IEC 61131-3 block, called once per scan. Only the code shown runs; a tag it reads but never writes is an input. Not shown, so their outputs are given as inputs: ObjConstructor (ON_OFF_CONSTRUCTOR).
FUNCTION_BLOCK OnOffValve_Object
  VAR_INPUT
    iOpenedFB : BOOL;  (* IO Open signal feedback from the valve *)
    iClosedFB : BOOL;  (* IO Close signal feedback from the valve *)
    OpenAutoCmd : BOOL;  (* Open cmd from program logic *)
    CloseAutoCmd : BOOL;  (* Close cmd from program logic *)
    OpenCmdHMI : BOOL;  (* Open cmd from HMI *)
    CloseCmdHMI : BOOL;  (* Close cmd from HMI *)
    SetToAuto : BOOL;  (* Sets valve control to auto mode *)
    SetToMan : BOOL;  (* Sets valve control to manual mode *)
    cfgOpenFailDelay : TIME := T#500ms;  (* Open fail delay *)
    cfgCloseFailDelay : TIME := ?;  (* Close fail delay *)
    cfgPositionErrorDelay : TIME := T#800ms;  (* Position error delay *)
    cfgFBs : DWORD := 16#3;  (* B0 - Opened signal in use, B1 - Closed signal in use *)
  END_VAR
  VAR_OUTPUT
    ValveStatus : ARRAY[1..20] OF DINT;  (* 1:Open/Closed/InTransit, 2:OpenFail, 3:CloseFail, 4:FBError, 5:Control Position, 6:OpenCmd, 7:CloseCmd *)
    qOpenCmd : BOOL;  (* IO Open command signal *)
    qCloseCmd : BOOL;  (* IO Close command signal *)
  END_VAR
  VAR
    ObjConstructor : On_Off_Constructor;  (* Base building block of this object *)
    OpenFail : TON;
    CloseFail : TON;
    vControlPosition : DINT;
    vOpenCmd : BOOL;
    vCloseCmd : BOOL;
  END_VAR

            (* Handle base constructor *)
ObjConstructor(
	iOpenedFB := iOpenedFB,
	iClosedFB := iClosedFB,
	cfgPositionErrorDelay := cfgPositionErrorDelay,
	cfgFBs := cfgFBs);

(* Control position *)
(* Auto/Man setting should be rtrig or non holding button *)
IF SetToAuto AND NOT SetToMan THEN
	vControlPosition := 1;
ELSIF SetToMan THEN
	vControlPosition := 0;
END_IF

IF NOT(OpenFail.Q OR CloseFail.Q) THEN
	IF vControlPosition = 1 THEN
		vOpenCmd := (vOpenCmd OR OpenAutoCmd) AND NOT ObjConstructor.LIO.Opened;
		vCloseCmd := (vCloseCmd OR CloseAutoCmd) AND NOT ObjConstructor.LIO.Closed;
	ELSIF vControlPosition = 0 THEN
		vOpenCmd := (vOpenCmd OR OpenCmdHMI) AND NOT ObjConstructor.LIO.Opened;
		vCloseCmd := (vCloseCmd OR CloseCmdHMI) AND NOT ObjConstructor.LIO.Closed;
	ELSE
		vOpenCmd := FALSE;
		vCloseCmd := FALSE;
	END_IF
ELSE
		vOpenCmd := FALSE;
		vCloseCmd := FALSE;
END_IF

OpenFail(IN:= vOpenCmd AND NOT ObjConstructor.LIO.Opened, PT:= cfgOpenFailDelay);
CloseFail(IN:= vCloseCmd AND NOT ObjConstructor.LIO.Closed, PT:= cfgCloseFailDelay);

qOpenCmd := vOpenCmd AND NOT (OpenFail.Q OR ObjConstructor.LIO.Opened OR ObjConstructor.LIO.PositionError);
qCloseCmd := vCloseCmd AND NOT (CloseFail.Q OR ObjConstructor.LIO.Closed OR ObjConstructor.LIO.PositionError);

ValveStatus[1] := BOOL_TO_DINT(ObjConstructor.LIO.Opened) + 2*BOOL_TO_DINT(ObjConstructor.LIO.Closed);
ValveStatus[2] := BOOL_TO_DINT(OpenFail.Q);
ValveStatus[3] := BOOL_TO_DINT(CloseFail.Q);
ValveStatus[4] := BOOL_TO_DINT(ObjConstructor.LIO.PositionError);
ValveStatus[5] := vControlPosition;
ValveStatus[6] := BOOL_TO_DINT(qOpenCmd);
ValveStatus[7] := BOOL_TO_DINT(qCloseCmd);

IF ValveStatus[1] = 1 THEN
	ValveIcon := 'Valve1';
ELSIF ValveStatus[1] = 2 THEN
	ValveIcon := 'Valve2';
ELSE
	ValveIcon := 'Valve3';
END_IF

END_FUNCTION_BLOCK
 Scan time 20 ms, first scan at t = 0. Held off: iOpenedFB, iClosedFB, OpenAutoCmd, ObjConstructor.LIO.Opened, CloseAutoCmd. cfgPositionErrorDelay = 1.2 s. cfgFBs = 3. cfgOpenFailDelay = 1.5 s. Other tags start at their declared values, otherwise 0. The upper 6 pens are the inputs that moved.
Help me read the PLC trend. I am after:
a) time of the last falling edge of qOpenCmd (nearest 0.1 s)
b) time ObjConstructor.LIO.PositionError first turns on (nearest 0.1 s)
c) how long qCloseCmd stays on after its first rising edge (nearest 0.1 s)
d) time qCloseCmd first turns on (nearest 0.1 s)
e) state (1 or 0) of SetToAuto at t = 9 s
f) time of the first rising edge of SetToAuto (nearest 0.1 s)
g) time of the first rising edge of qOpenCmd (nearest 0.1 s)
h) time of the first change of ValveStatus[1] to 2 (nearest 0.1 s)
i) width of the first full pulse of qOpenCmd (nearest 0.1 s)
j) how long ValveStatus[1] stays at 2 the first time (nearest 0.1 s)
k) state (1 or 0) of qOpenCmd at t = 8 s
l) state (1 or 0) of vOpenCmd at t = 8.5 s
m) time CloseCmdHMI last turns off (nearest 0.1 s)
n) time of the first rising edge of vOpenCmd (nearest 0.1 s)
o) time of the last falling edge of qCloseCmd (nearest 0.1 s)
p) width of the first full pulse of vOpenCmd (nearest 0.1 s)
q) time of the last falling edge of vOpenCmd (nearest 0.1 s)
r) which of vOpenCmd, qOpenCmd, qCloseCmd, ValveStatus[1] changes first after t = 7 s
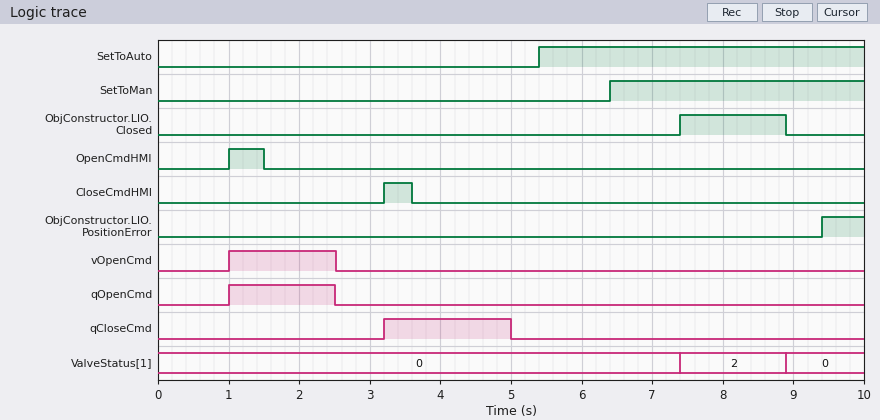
2.5 s
9.4 s
1.8 s
3.2 s
1
5.4 s
1.0 s
7.4 s
1.5 s
1.5 s
0
0
3.6 s
1.0 s
5.0 s
1.5 s
2.5 s
ValveStatus[1]
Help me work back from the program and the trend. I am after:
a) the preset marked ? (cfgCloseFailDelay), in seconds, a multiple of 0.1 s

1.8 s
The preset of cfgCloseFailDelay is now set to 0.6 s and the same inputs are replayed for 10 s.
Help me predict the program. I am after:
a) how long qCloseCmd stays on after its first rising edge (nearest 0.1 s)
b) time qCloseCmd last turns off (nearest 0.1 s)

0.6 s
3.8 s
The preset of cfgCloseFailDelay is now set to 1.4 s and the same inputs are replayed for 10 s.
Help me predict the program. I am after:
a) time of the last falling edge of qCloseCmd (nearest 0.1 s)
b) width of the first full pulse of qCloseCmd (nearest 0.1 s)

4.6 s
1.4 s
